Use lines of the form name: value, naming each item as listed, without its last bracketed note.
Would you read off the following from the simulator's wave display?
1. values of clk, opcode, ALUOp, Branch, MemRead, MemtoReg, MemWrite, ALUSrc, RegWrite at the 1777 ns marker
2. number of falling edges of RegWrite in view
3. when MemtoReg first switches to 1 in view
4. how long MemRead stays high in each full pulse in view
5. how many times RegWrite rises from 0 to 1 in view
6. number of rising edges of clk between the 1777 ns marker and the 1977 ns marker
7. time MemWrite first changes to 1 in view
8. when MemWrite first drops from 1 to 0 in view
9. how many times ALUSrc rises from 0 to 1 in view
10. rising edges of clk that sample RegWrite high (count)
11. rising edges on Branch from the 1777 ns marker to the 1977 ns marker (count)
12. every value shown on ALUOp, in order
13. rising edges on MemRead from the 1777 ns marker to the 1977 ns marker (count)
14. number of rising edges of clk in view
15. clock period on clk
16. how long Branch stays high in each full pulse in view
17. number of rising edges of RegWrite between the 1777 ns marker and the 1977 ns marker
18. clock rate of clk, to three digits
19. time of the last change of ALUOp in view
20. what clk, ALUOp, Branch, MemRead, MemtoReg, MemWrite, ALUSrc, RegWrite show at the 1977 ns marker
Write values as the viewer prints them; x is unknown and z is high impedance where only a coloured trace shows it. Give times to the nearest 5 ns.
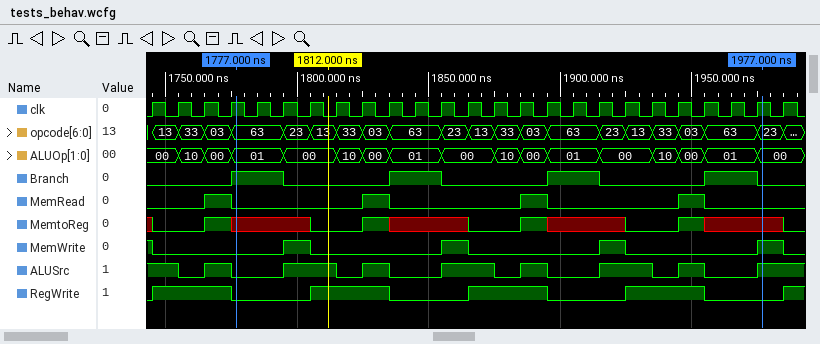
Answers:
values of clk, opcode, ALUOp, Branch, MemRead, MemtoReg, MemWrite, ALUSrc, RegWrite at the 1777 ns marker: clk=1, opcode=63, ALUOp=01, Branch=1, MemRead=0, MemtoReg=x, MemWrite=0, ALUSrc=0, RegWrite=0
number of falling edges of RegWrite in view: 4
when MemtoReg first switches to 1 in view: 1765 ns
how long MemRead stays high in each full pulse in view: 10 ns, 10 ns, 10 ns, 10 ns
how many times RegWrite rises from 0 to 1 in view: 5
number of rising edges of clk between the 1777 ns marker and the 1977 ns marker: 20
time MemWrite first changes to 1 in view: 1795 ns
when MemWrite first drops from 1 to 0 in view: 1745 ns
how many times ALUSrc rises from 0 to 1 in view: 8
rising edges of clk that sample RegWrite high: 12
rising edges on Branch from the 1777 ns marker to the 1977 ns marker: 3
every value shown on ALUOp, in order: 00, 10, 00, 01, 00, 10, 00, 01, 00, 10, 00, 01, 00, 10, 00, 01, 00
rising edges on MemRead from the 1777 ns marker to the 1977 ns marker: 3
number of rising edges of clk in view: 25
clock period on clk: 10 ns
how long Branch stays high in each full pulse in view: 20 ns, 20 ns, 20 ns, 20 ns
number of rising edges of RegWrite between the 1777 ns marker and the 1977 ns marker: 3
clock rate of clk, to three digits: 100 MHz
time of the last change of ALUOp in view: 1975 ns
what clk, ALUOp, Branch, MemRead, MemtoReg, MemWrite, ALUSrc, RegWrite show at the 1977 ns marker: clk=1, ALUOp=00, Branch=0, MemRead=0, MemtoReg=x, MemWrite=1, ALUSrc=1, RegWrite=0
